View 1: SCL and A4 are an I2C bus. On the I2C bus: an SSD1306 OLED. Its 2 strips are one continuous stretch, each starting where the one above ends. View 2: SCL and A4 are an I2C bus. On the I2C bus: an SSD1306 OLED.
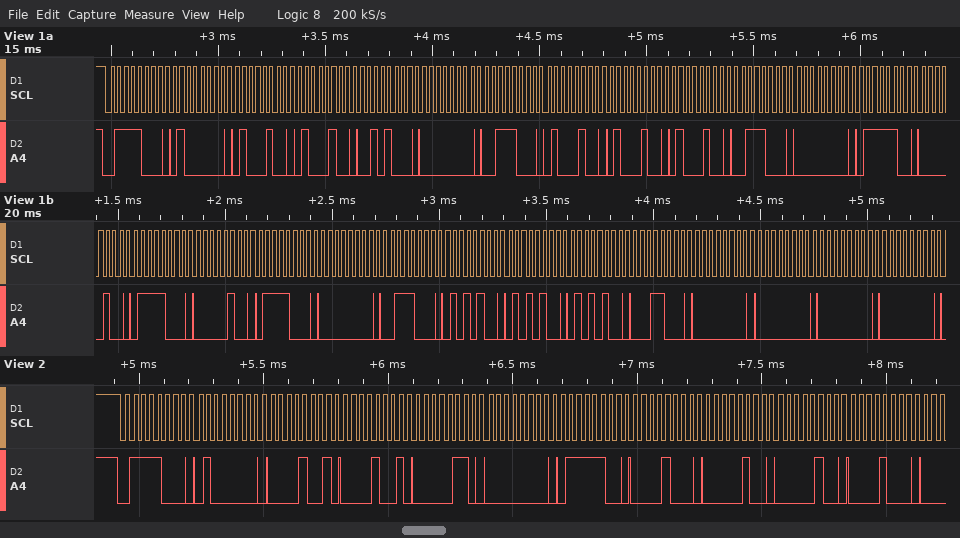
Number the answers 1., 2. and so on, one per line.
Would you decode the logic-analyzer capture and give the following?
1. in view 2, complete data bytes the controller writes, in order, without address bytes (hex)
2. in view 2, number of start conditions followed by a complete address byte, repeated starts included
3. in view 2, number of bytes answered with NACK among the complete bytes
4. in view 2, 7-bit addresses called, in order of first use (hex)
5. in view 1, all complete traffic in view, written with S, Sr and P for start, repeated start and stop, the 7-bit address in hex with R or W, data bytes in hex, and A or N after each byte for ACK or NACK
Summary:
1. 40 09 09 06 00 7C 08 04 04 08
2. 1
3. 0
4. 0x3C
5. S 3CW A 40 A 44 A 44 A 28 A 00 A 38 A 44 A 44 A 44 A 38 A 00 A 7C A 04 A 78 A 04 A 78 A 00 A 38 A 54 A 54 A 54 A 18 A 00 A 00 A 00 A 00 A
